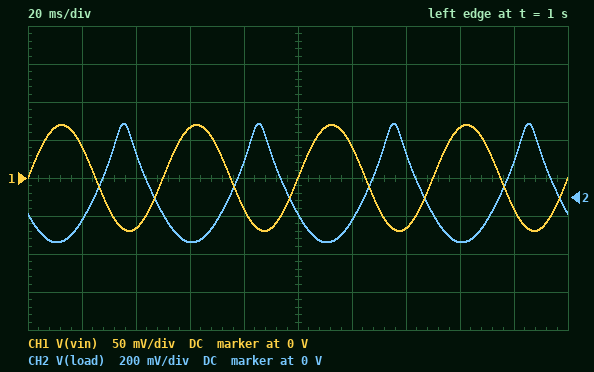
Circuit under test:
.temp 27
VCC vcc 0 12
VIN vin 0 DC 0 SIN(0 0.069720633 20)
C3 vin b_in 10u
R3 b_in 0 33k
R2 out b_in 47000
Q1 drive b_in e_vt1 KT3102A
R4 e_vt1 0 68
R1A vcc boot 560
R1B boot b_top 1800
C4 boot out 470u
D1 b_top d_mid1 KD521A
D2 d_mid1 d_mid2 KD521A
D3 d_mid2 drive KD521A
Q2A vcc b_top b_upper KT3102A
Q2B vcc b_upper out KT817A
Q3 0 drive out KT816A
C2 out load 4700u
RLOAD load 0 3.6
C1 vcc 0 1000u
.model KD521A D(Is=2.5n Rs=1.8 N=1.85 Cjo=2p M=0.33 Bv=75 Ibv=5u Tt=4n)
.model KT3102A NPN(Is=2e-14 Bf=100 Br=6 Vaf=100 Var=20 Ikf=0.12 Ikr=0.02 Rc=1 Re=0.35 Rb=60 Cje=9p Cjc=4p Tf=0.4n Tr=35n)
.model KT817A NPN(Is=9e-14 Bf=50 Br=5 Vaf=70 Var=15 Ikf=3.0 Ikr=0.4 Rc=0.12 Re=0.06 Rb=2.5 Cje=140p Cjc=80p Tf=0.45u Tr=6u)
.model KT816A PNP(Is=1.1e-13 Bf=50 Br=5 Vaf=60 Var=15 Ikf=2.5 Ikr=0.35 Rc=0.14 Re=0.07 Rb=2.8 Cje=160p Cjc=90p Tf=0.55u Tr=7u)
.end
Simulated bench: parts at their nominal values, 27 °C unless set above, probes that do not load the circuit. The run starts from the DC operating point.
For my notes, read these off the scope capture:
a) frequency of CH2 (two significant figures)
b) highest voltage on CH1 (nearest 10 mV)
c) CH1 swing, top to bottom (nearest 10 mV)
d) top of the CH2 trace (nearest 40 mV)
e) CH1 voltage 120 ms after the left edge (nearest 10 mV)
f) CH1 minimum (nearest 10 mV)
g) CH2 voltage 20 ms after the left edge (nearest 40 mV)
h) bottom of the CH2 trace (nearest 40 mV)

20 Hz
70 mV
140 mV
400 mV
40 mV
-70 mV
-120 mV
-240 mV
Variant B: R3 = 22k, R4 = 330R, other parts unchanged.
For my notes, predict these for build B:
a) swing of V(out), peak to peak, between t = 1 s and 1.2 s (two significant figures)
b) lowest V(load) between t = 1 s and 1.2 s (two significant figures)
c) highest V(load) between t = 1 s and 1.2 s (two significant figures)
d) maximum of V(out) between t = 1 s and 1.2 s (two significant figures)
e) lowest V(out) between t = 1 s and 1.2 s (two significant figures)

120 mV
-53 mV
59 mV
5.9 V
5.8 V
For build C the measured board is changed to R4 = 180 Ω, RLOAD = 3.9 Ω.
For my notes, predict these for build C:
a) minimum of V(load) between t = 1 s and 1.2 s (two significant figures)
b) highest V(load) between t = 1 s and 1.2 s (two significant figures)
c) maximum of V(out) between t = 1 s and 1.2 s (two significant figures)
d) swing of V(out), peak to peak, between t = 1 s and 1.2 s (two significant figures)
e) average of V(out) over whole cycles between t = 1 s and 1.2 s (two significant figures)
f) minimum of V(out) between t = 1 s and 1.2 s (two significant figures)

-100 mV
120 mV
4.7 V
240 mV
4.6 V
4.5 V
